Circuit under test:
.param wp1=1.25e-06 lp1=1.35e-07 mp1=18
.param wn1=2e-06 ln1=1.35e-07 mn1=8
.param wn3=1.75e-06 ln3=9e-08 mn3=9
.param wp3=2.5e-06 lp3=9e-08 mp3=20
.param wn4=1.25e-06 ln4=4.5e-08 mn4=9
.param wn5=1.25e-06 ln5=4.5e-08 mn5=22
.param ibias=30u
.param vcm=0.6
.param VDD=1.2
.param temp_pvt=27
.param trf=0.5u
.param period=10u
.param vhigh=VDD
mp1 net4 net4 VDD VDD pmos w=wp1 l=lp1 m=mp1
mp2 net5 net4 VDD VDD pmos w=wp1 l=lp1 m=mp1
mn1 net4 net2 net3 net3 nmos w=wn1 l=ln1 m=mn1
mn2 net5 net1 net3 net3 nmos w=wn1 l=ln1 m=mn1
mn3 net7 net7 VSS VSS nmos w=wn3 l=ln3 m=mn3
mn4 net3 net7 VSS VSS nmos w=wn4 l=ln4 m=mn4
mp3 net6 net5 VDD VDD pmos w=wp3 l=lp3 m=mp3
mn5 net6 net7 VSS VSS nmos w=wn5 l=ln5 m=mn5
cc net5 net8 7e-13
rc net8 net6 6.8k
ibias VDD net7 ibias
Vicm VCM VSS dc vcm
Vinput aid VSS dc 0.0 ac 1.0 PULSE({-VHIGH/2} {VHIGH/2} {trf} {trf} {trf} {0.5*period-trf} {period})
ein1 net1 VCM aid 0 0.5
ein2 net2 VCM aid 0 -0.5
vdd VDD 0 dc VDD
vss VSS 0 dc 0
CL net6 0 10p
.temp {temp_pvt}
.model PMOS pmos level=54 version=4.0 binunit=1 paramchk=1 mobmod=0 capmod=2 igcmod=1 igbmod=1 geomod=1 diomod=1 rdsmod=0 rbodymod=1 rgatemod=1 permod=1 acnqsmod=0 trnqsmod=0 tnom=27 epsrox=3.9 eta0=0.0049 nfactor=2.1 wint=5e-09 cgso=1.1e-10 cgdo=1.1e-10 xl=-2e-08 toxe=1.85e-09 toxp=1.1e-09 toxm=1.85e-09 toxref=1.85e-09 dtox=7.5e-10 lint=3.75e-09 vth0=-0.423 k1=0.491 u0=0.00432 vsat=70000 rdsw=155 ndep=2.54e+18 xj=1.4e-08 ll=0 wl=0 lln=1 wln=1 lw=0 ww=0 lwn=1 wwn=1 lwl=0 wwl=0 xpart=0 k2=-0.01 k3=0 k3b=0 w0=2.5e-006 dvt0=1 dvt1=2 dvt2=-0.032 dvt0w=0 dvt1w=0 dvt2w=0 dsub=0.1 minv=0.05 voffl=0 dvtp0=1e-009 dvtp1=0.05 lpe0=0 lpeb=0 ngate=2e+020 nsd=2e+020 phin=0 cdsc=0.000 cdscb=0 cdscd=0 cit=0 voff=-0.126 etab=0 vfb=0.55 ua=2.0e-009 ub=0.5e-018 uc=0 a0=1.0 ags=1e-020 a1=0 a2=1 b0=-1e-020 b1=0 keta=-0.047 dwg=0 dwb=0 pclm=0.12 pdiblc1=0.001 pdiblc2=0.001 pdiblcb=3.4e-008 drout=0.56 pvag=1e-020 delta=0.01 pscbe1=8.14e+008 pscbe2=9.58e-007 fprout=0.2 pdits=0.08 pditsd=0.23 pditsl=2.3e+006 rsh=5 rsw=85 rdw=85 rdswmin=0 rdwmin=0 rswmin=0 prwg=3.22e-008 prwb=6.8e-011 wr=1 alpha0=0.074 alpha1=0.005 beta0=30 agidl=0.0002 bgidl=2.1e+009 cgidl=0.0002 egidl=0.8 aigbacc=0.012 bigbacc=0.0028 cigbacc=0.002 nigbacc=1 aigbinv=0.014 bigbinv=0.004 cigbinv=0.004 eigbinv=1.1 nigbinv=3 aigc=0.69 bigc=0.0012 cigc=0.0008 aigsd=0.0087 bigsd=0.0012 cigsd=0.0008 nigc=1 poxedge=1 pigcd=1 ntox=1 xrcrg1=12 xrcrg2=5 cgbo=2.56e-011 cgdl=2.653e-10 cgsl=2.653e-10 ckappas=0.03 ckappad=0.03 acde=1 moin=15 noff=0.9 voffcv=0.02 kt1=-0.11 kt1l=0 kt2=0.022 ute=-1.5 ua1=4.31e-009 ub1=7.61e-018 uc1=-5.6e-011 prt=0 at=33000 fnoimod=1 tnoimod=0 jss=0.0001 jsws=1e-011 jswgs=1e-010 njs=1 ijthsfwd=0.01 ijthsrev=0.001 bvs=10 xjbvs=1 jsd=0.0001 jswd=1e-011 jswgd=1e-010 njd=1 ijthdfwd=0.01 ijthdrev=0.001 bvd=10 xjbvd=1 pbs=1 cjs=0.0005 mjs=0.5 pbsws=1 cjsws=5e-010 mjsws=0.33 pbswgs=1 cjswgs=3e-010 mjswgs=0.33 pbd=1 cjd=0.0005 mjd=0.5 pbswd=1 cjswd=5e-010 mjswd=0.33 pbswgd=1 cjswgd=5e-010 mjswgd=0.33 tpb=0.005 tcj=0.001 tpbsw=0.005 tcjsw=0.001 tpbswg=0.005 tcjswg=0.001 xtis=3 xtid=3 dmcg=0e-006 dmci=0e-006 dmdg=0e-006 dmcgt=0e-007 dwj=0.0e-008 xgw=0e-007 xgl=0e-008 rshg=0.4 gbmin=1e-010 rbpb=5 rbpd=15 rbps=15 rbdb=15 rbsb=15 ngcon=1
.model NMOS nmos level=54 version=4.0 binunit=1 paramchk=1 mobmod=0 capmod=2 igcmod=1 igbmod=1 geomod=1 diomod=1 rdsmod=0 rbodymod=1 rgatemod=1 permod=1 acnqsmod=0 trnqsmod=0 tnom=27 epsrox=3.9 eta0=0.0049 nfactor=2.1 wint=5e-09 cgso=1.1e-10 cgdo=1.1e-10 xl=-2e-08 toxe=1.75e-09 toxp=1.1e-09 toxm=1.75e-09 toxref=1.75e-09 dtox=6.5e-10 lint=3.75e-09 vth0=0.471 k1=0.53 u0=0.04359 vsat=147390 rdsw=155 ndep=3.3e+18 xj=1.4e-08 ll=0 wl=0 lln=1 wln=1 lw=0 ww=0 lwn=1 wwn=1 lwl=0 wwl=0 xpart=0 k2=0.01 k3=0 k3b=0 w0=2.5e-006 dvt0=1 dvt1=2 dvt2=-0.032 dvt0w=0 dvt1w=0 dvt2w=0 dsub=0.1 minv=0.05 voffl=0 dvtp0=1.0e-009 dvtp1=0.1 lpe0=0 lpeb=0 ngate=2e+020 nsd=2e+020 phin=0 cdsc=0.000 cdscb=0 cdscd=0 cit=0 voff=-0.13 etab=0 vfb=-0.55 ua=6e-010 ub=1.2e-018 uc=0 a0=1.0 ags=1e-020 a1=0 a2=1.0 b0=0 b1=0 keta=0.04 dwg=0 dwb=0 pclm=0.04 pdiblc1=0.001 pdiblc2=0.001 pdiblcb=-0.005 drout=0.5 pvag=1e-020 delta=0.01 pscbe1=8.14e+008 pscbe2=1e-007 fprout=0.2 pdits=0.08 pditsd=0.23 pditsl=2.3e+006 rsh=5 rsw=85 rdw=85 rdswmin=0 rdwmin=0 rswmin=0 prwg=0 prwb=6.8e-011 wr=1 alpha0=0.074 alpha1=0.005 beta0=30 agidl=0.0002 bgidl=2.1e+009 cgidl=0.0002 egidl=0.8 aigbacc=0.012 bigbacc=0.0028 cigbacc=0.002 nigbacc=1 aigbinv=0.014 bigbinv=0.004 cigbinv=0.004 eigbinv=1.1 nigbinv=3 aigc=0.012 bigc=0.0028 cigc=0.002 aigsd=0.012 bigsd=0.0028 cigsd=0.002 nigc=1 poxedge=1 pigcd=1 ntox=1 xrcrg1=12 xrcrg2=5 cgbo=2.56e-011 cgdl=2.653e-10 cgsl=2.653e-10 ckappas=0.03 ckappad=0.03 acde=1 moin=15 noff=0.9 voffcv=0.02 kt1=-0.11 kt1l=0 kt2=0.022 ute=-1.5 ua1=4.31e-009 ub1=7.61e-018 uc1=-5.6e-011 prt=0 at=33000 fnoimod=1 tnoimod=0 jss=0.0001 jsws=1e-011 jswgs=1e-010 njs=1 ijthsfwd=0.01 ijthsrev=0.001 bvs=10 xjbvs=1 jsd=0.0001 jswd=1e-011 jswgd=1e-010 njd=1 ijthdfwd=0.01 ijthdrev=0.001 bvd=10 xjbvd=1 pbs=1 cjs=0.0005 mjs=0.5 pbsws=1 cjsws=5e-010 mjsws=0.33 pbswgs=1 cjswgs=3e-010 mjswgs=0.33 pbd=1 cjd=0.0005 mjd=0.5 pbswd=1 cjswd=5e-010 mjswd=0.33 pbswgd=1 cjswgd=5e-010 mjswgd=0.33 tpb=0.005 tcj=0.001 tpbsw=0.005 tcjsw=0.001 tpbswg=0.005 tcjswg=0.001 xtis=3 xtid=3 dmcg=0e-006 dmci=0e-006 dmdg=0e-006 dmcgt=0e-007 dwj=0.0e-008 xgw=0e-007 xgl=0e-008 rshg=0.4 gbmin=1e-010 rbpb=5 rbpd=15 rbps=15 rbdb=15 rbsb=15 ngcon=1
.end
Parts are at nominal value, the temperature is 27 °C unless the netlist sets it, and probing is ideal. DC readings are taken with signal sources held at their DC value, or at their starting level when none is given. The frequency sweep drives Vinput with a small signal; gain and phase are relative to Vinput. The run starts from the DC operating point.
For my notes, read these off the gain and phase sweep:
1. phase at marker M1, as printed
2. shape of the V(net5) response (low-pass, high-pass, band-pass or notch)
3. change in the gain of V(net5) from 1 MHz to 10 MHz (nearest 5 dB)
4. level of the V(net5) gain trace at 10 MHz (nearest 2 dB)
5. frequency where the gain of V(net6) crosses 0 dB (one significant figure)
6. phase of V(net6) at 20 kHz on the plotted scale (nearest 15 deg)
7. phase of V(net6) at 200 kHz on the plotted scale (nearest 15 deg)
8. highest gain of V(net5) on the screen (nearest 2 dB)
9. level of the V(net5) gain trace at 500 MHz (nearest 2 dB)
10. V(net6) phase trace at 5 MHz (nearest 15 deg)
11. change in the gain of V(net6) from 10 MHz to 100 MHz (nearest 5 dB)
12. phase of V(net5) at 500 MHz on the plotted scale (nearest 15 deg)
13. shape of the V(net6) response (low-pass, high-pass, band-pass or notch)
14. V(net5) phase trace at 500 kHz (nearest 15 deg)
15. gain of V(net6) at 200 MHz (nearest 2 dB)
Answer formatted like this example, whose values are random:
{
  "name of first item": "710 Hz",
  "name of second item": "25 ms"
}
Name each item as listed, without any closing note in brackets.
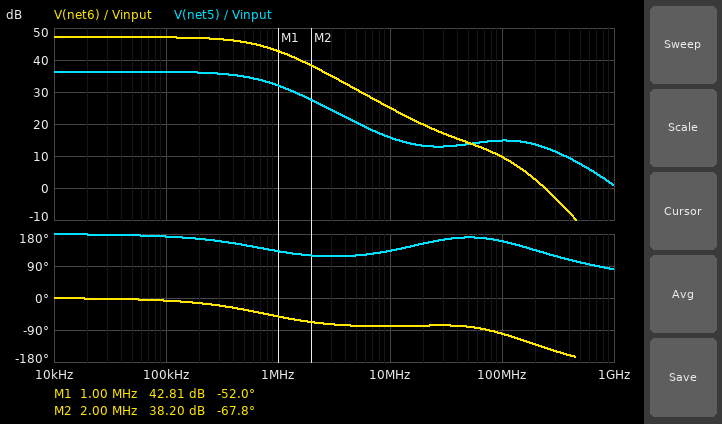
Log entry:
{
  "phase at marker M1, as printed": "-52.0 deg",
  "shape of the V(net5) response": "low-pass",
  "change in the gain of V(net5) from 1 MHz to 10 MHz": "-15 dB",
  "level of the V(net5) gain trace at 10 MHz": "16 dB",
  "frequency where the gain of V(net6) crosses 0 dB": "200 MHz",
  "phase of V(net6) at 20 kHz on the plotted scale": "0 deg",
  "phase of V(net6) at 200 kHz on the plotted scale": "-15 deg",
  "highest gain of V(net5) on the screen": "36 dB",
  "level of the V(net5) gain trace at 500 MHz": "8 dB",
  "V(net6) phase trace at 5 MHz": "-75 deg",
  "change in the gain of V(net6) from 10 MHz to 100 MHz": "-15 dB",
  "phase of V(net5) at 500 MHz on the plotted scale": "105 deg",
  "shape of the V(net6) response": "low-pass",
  "V(net5) phase trace at 500 kHz": "150 deg",
  "gain of V(net6) at 200 MHz": "2 dB"
}
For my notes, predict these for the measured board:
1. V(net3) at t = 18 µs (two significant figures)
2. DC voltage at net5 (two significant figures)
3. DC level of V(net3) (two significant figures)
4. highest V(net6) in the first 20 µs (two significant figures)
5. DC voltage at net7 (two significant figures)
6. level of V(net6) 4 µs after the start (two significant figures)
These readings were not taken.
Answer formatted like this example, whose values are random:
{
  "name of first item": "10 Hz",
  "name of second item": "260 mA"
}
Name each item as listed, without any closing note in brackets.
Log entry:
{
  "V(net3) at t = 18 µs": "390 mV",
  "DC voltage at net5": "690 mV",
  "DC level of V(net3)": "170 mV",
  "highest V(net6) in the first 20 µs": "1.0 V",
  "DC voltage at net7": "360 mV",
  "level of V(net6) 4 µs after the start": "1.0 V"
}
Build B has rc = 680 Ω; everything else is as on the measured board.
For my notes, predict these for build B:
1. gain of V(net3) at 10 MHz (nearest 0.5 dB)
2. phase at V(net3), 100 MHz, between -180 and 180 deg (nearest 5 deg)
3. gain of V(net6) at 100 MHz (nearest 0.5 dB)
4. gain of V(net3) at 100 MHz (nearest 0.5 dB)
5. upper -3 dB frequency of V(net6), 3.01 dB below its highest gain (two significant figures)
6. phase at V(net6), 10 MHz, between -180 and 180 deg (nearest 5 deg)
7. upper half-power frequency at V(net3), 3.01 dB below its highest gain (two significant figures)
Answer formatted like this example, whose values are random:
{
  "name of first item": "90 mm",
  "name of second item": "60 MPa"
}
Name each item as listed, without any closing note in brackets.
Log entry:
{
  "gain of V(net3) at 10 MHz": "-30.0 dB",
  "phase at V(net3), 100 MHz, between -180 and 180 deg": "130 deg",
  "gain of V(net6) at 100 MHz": "0.5 dB",
  "gain of V(net3) at 100 MHz": "-35.5 dB",
  "upper -3 dB frequency of V(net6), 3.01 dB below its highest gain": "780 kHz",
  "phase at V(net6), 10 MHz, between -180 and 180 deg": "-95 deg",
  "upper half-power frequency at V(net3), 3.01 dB below its highest gain": "790 kHz"
}
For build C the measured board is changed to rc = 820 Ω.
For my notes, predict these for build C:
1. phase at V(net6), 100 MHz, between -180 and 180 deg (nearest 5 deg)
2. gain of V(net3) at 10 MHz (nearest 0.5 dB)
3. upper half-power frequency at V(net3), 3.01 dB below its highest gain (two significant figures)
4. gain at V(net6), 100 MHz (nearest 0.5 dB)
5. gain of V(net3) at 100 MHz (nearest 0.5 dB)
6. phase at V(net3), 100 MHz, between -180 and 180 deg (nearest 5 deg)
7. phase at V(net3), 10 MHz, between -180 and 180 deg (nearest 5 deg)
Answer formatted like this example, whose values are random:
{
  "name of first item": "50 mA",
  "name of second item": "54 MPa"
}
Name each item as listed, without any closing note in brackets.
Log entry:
{
  "phase at V(net6), 100 MHz, between -180 and 180 deg": "-135 deg",
  "gain of V(net3) at 10 MHz": "-30.0 dB",
  "upper half-power frequency at V(net3), 3.01 dB below its highest gain": "790 kHz",
  "gain at V(net6), 100 MHz": "0.5 dB",
  "gain of V(net3) at 100 MHz": "-35.5 dB",
  "phase at V(net3), 100 MHz, between -180 and 180 deg": "130 deg",
  "phase at V(net3), 10 MHz, between -180 and 180 deg": "145 deg"
}
